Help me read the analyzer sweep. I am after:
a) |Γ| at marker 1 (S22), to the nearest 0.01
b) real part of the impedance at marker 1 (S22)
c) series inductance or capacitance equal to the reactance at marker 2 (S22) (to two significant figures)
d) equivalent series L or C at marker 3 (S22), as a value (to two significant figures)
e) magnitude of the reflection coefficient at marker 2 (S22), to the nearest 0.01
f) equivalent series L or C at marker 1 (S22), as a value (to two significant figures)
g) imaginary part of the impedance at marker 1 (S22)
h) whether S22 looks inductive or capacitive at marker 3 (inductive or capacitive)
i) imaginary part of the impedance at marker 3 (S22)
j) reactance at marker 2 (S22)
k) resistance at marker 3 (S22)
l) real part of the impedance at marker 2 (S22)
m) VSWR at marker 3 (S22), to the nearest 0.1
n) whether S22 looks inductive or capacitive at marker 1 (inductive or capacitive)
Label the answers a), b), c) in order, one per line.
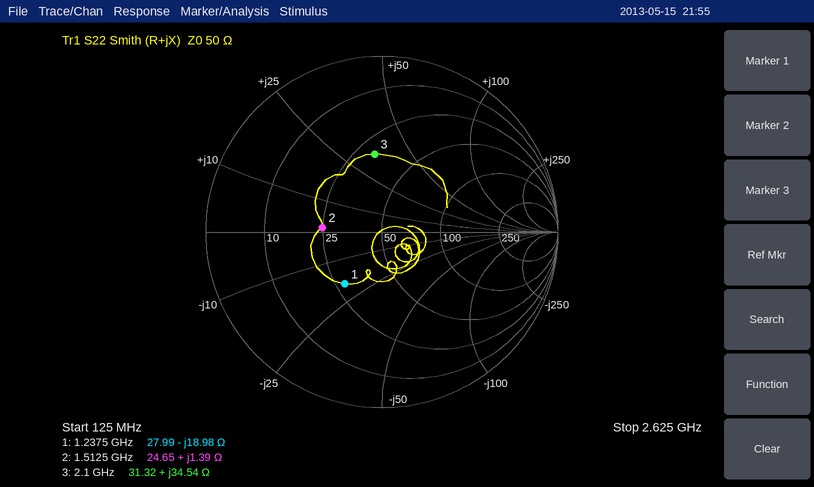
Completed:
a) 0.36
b) 27.99 Ω
c) 150 pH
d) 2.6 nH
e) 0.34
f) 6.8 pF
g) -18.98 Ω
h) inductive
i) +34.54 Ω
j) +1.39 Ω
k) 31.32 Ω
l) 24.65 Ω
m) 2.6
n) capacitive
